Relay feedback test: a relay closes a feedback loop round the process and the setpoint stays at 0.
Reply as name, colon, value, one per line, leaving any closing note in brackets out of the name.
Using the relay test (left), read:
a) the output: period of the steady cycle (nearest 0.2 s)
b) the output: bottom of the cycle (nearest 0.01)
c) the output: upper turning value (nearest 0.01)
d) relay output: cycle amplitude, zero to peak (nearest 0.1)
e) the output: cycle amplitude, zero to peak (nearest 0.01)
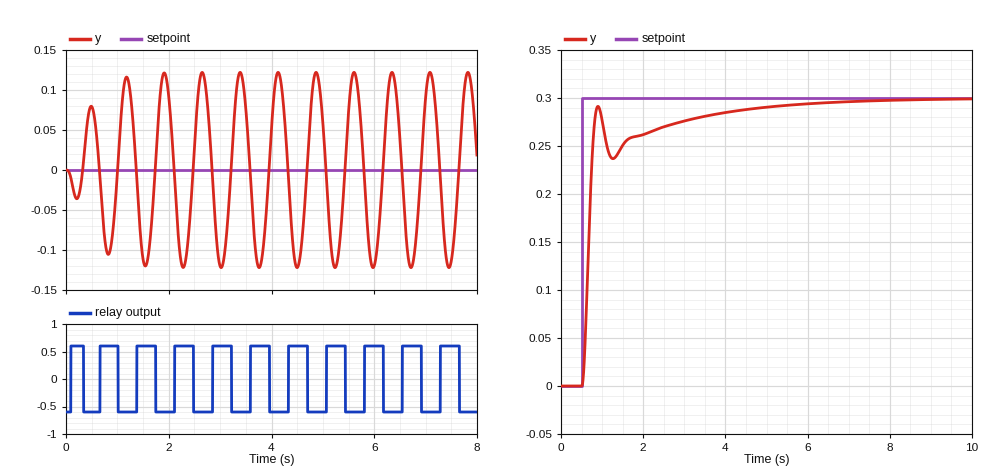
the output: period of the steady cycle: 0.8 s
the output: bottom of the cycle: -0.12
the output: upper turning value: 0.12
relay output: cycle amplitude, zero to peak: 0.6
the output: cycle amplitude, zero to peak: 0.12
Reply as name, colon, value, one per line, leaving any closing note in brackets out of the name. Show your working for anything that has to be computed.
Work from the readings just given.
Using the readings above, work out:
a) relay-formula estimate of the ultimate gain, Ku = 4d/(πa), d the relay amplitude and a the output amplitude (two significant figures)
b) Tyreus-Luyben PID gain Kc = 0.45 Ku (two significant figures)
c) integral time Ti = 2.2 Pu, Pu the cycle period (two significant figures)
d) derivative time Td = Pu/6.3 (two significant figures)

relay-formula estimate of the ultimate gain, Ku = 4d/(πa), d the relay amplitude and a the output amplitude: 4 × 0.6 / (π × 0.12) = 6.4
Tyreus-Luyben PID gain Kc = 0.45 Ku: 0.45 × 6.4 = 2.9
integral time Ti = 2.2 Pu, Pu the cycle period: 2.2 × 0.8 = 1.8 s
derivative time Td = Pu/6.3: 0.8 / 6.3 = 0.13 s
